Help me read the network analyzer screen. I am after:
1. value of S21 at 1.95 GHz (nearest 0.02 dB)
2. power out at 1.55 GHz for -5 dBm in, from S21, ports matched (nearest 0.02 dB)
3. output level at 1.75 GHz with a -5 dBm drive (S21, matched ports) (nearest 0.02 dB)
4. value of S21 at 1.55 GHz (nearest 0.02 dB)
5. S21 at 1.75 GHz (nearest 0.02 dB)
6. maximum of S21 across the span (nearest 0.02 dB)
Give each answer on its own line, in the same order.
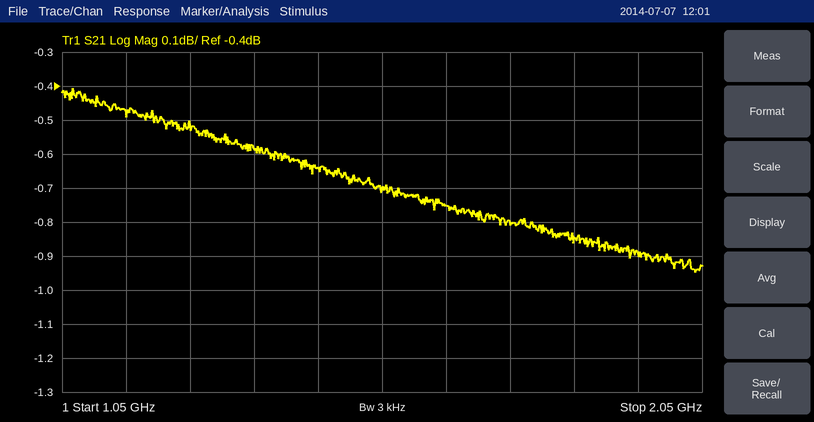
-0.90 dB
-5.70 dBm
-5.80 dBm
-0.70 dB
-0.80 dB
-0.40 dB
